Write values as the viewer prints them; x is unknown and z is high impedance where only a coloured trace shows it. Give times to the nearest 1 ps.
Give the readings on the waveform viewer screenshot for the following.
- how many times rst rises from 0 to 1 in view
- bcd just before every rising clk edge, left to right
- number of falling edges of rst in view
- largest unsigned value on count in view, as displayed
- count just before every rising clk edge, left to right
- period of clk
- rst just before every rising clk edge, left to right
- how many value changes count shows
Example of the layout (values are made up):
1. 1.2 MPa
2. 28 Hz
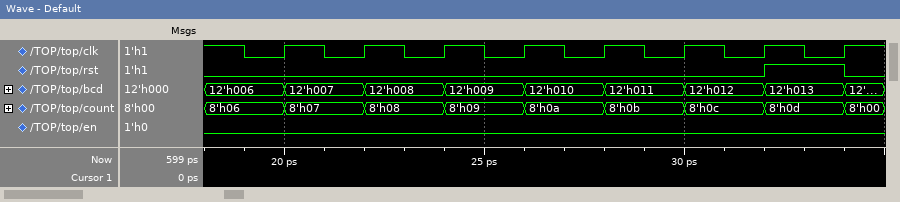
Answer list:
1. 1
2. 12'h006, 12'h007, 12'h008, 12'h009, 12'h010, 12'h011, 12'h012, 12'h013
3. 1
4. 8'h0d
5. 8'h06, 8'h07, 8'h08, 8'h09, 8'h0a, 8'h0b, 8'h0c, 8'h0d
6. 2 ps
7. 0 0 0 0 0 0 0 1
8. 8
